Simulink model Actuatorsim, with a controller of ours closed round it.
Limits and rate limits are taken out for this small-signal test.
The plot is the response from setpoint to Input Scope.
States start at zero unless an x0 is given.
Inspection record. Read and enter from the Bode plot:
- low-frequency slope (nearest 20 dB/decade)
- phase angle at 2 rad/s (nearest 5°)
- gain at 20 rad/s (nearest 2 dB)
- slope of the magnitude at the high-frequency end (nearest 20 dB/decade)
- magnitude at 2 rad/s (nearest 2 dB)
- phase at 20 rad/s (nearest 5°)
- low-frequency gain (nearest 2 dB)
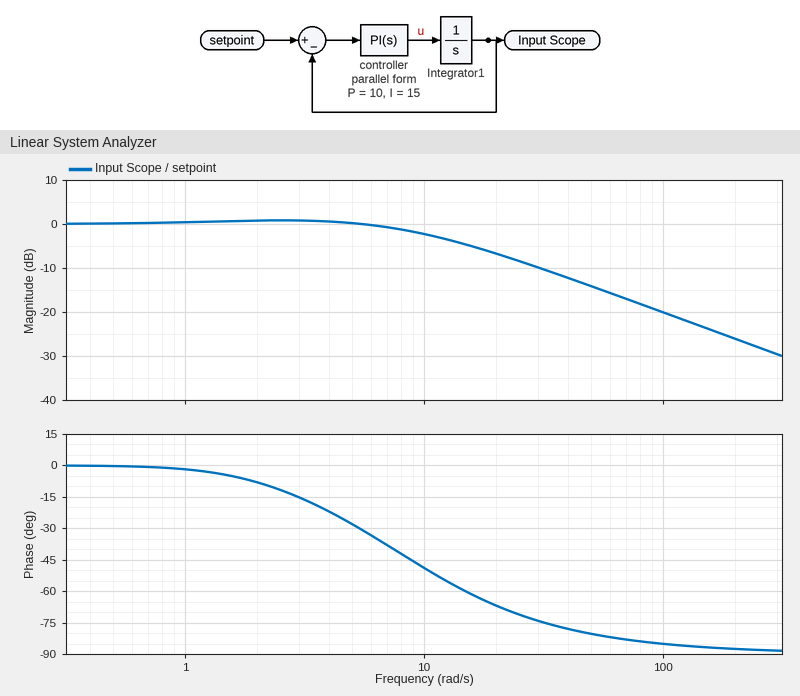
0 dB/decade
-10°
-6 dB
-20 dB/decade
0 dB
-65°
0 dB
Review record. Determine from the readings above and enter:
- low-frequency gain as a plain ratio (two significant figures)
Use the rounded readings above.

1.0
